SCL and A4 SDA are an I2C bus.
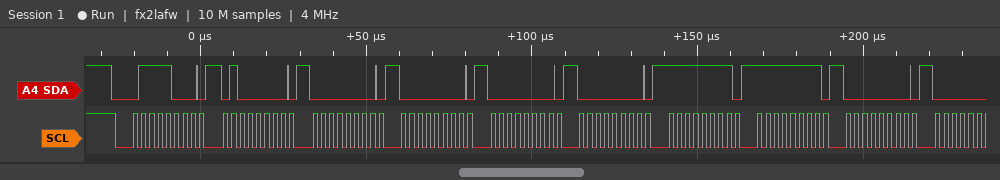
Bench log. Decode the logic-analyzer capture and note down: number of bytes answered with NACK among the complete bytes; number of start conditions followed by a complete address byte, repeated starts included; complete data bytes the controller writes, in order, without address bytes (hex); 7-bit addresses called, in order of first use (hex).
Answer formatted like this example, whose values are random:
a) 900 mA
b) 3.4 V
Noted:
a) 0
b) 1
c) 40 00 00 00 00 FF FF 00
d) 0x3C
